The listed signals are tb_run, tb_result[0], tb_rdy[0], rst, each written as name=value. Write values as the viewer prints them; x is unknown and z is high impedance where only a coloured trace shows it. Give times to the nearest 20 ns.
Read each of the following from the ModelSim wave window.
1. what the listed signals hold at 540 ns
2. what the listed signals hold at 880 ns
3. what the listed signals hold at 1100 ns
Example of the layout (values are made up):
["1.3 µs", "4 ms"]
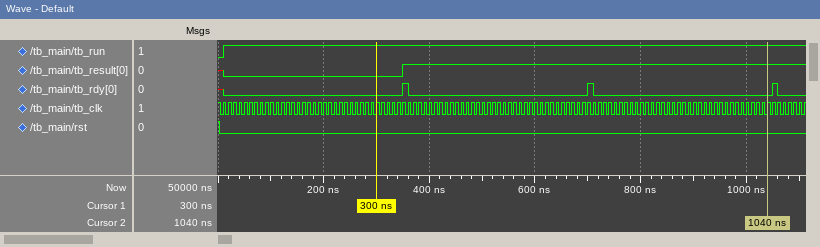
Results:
["tb_run=1, tb_result[0]=1, tb_rdy[0]=0, rst=0", "tb_run=1, tb_result[0]=1, tb_rdy[0]=0, rst=0", "tb_run=1, tb_result[0]=1, tb_rdy[0]=0, rst=0"]
